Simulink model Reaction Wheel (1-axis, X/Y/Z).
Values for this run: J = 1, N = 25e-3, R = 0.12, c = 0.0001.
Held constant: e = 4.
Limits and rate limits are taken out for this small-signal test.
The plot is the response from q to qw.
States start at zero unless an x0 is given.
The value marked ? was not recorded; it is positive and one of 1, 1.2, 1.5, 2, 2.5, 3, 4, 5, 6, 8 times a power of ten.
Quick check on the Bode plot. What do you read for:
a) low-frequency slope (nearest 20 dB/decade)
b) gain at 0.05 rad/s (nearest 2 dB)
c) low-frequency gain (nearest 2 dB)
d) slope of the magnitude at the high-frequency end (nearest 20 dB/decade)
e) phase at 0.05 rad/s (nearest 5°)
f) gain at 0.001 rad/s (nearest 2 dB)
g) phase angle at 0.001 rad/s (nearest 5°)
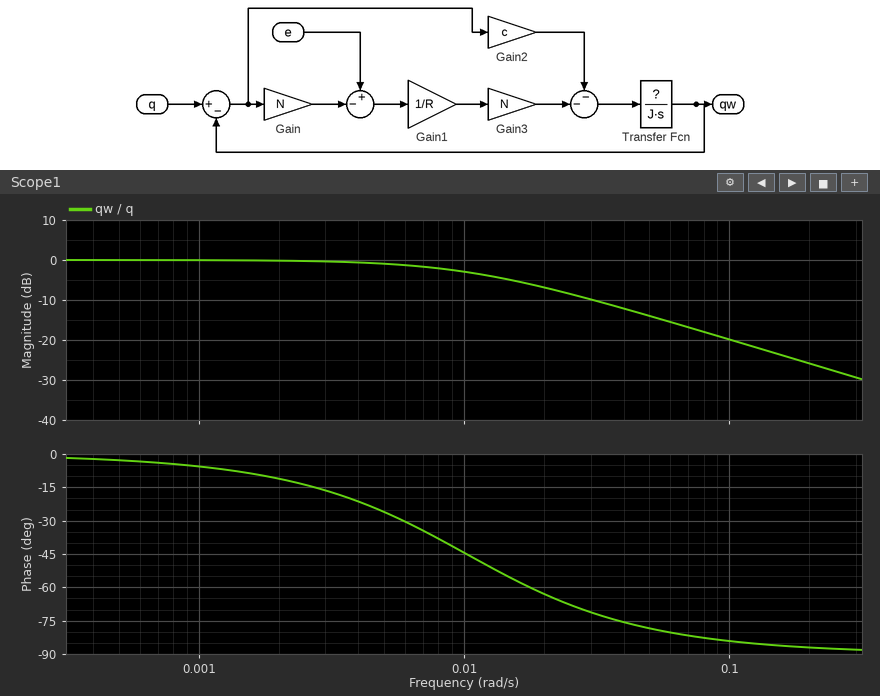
0 dB/decade
-14 dB
0 dB
-20 dB/decade
-80°
0 dB
-5°
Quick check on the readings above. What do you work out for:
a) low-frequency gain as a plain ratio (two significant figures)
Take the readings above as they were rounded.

1.0
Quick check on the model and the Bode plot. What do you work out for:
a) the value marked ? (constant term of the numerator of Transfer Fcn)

2
